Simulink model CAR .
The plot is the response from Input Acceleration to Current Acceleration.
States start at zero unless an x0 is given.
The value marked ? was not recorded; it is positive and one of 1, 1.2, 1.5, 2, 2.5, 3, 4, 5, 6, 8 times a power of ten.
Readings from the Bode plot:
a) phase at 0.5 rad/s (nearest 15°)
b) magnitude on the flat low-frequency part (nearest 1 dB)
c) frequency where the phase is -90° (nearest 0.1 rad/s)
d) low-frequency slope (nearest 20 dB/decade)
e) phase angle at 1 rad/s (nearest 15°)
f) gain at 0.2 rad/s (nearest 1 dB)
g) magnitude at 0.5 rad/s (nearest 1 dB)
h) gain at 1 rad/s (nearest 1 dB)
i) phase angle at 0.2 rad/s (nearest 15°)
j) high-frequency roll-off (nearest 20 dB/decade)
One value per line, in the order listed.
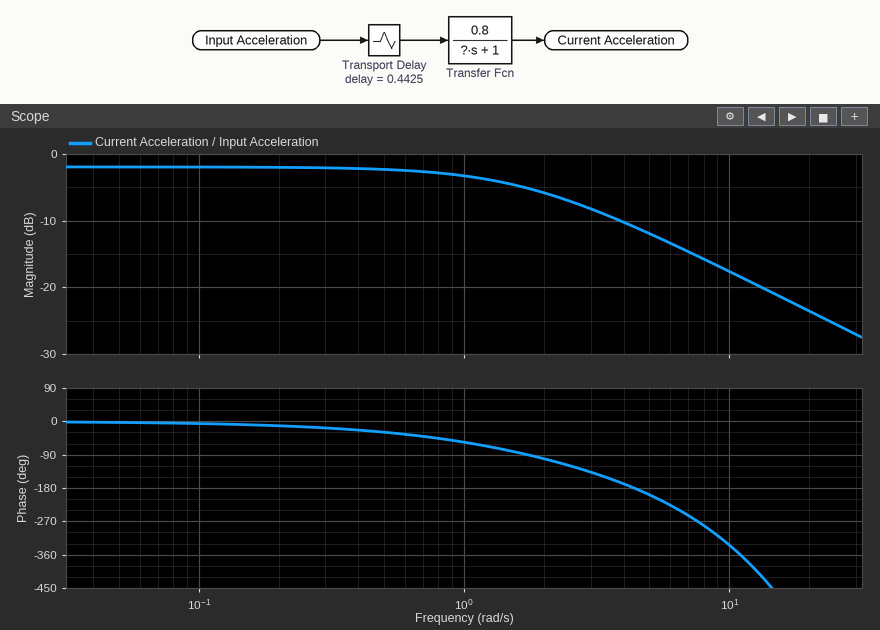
-30°
-2 dB
1.7 rad/s
0 dB/decade
-60°
-2 dB
-2 dB
-3 dB
-15°
-20 dB/decade
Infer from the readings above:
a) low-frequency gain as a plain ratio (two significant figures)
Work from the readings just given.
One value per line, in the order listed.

0.79
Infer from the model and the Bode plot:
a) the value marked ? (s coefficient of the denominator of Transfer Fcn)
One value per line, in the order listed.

0.6
